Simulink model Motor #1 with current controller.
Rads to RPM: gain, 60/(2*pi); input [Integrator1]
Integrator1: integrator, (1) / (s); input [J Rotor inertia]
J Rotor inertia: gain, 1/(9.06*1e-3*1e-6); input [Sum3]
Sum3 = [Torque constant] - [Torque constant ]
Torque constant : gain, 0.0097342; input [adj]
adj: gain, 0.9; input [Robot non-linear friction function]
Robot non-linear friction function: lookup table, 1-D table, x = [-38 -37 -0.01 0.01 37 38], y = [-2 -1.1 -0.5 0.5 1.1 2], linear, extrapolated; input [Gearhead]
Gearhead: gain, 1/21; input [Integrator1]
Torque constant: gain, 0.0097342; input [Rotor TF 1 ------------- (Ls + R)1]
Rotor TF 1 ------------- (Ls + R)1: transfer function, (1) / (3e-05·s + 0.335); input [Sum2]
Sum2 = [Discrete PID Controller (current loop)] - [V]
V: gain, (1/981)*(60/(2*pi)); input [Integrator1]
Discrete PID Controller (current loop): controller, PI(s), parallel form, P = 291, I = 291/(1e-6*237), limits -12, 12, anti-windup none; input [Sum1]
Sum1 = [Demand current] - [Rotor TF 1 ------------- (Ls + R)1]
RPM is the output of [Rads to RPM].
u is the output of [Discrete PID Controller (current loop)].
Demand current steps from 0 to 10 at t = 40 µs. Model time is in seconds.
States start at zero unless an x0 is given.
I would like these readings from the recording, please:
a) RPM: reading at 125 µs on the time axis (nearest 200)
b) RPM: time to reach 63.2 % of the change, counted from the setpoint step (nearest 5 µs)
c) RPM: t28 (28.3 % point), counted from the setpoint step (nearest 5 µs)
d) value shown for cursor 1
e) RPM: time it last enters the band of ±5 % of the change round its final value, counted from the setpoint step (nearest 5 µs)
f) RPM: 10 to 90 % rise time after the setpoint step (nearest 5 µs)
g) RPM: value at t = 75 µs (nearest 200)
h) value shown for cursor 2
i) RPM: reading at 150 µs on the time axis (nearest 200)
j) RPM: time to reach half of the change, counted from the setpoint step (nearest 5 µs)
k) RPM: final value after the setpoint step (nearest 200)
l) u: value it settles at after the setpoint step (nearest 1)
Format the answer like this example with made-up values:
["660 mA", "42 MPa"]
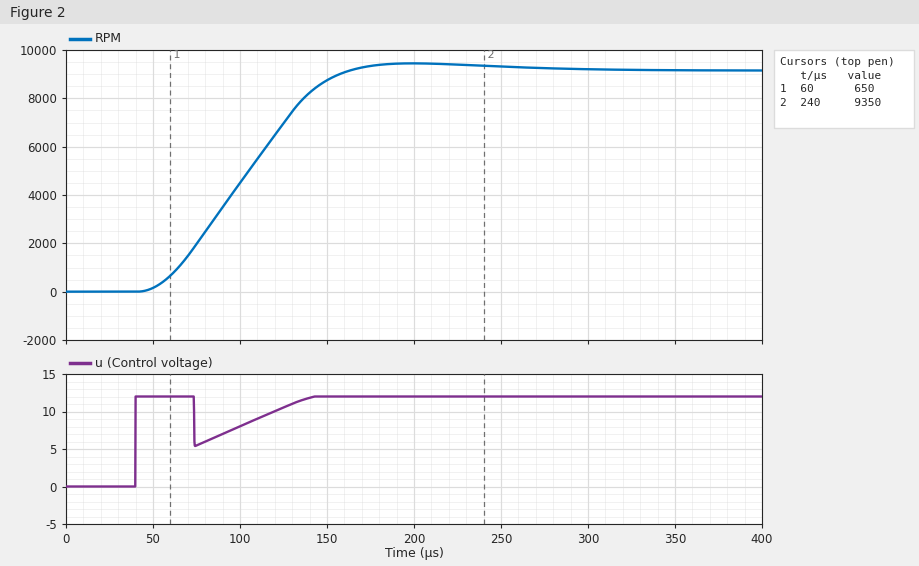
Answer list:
["7000", "75 µs", "40 µs", "650", "110 µs", "75 µs", "2000", "9350", "8800", "60 µs", "9200", "12"]
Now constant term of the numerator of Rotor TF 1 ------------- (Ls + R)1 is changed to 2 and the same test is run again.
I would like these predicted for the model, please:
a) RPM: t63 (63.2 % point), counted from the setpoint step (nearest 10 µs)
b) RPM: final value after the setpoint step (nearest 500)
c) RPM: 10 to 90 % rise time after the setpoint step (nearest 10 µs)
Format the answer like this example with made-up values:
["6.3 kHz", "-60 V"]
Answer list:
["70 µs", "9500", "90 µs"]
